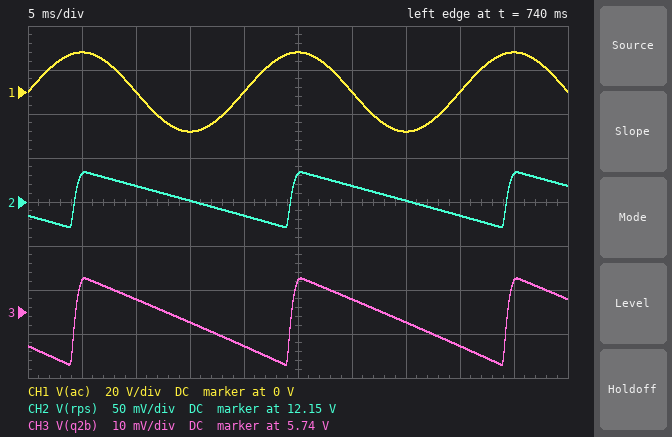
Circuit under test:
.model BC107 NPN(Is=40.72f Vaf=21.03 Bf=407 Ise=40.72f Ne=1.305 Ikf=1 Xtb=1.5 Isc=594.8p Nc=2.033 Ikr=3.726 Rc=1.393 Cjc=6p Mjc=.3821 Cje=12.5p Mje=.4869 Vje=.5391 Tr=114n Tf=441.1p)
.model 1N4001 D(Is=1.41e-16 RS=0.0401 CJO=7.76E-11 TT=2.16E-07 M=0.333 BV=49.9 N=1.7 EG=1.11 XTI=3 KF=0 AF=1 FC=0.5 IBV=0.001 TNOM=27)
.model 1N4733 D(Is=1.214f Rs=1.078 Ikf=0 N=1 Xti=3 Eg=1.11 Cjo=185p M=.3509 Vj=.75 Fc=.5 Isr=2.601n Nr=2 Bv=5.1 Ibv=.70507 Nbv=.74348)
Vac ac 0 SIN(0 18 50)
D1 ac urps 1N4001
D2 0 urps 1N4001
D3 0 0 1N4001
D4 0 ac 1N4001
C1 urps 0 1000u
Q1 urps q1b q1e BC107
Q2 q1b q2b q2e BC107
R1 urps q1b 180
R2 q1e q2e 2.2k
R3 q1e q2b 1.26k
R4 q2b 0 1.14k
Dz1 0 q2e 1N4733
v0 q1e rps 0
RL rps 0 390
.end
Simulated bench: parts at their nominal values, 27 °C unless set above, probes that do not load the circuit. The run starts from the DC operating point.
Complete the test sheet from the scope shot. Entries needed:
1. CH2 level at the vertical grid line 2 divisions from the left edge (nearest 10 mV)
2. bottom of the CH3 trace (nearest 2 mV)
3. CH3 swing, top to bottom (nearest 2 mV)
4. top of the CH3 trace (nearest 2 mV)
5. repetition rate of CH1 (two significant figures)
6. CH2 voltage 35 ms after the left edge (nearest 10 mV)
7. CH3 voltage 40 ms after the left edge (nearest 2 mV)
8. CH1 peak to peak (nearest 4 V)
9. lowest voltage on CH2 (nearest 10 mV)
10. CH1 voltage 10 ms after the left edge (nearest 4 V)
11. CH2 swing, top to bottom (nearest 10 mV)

12.17 V
5.728 V
20 mV
5.748 V
50 Hz
12.15 V
5.732 V
36 V
12.12 V
0 V
60 mV
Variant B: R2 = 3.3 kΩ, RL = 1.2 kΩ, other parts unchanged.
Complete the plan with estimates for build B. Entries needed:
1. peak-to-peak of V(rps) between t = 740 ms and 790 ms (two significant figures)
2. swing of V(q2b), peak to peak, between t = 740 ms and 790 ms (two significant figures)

39 mV
12 mV
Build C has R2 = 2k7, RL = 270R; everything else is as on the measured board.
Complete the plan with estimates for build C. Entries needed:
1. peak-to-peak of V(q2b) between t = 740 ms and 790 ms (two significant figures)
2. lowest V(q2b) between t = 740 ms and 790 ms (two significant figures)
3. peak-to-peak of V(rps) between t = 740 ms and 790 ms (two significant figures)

25 mV
5.7 V
78 mV
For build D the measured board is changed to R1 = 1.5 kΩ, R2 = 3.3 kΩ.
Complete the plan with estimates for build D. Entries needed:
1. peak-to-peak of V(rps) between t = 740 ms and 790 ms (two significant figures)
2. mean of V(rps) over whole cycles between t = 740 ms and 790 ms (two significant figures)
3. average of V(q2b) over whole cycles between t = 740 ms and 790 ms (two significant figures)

20 mV
12 V
5.6 V
